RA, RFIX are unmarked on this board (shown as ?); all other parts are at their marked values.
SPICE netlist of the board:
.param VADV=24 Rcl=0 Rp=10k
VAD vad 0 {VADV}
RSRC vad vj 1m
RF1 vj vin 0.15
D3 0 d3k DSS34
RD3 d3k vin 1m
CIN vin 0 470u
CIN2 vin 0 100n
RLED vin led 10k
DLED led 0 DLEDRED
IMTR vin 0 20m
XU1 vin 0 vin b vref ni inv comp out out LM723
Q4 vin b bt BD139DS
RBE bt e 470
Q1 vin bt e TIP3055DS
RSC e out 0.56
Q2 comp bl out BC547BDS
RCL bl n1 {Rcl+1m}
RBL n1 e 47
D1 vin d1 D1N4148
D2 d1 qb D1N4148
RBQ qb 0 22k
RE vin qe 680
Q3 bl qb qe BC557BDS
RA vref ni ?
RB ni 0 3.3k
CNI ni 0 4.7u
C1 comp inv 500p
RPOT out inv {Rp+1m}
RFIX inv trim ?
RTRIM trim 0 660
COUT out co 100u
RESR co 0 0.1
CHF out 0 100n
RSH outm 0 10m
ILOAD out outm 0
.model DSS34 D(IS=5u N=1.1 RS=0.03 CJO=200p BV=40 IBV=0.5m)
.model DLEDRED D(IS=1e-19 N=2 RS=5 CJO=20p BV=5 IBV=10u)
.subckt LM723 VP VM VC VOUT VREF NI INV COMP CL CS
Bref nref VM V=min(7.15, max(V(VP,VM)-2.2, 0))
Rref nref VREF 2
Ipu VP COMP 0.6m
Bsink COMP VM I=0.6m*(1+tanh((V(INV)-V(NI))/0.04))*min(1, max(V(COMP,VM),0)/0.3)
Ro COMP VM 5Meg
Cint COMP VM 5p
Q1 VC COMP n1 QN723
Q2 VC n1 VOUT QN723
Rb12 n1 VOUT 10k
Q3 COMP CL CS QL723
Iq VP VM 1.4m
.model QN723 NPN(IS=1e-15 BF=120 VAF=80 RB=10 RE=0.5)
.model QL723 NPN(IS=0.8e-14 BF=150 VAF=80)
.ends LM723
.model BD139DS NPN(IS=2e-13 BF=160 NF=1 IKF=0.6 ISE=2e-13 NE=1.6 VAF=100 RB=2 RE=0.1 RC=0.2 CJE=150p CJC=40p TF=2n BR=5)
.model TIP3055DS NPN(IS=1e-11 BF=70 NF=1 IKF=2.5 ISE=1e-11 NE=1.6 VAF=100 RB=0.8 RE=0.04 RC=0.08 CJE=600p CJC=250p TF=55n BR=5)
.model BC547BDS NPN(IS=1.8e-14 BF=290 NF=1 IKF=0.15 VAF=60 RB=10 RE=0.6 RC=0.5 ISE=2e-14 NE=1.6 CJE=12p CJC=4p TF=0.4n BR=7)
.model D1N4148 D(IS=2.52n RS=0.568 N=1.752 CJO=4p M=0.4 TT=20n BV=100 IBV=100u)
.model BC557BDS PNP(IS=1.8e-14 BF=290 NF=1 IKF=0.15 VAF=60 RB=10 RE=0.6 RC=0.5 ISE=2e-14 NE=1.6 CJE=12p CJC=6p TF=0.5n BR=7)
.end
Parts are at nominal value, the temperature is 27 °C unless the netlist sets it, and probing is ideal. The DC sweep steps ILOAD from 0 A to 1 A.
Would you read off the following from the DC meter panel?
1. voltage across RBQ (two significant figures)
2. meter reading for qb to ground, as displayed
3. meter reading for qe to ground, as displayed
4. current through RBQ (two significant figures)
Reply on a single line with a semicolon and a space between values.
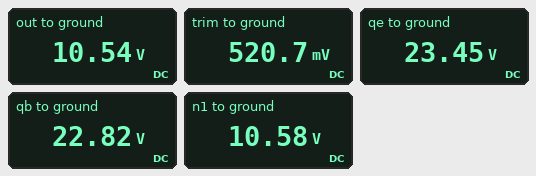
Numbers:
23 V; 22.82 V; 23.45 V; 1.0 mA
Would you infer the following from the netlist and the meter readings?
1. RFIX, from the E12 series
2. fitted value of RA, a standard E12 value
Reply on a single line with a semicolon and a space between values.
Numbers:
2.7 kΩ; 5.6 kΩ
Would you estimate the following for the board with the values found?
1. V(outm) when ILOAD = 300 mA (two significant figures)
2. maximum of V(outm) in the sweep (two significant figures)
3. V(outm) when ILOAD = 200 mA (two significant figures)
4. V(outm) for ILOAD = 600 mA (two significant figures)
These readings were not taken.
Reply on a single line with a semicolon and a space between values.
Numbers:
3.0 mV; 10 mV; 2.0 mV; 6.0 mV
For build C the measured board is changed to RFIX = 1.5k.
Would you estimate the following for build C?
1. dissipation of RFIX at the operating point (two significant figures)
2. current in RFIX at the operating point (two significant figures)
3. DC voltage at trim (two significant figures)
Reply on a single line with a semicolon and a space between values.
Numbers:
2.3 mW; 1.2 mA; 810 mV
